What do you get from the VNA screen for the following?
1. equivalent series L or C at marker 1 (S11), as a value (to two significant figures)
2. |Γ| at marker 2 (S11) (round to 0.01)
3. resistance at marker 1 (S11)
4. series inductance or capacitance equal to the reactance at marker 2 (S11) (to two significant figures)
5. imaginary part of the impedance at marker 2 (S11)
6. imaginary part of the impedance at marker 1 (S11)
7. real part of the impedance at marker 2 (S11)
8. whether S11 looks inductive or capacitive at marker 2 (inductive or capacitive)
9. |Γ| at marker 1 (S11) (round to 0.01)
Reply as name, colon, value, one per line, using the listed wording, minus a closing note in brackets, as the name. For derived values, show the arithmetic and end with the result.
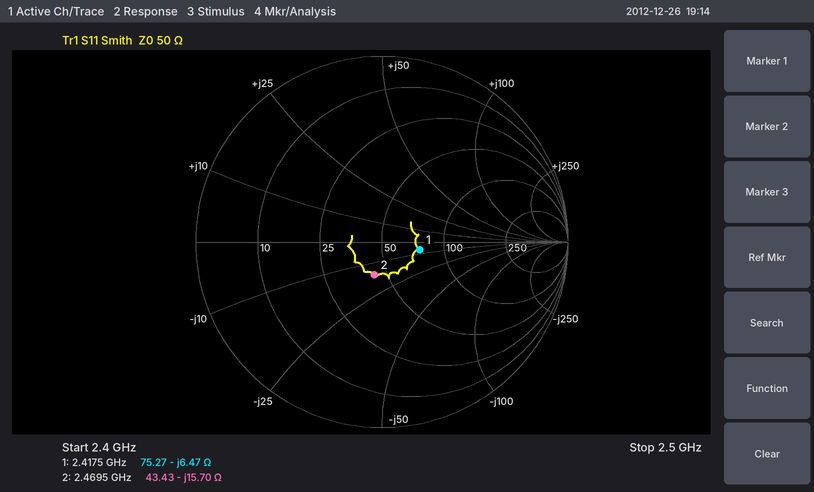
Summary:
equivalent series L or C at marker 1 (S11), as a value: C = 1/(2π × 2.4175 GHz × 6.47 Ω) ≈ 10 pF
|Γ| at marker 2 (S11): 0.18
resistance at marker 1: 75.27 Ω
series inductance or capacitance equal to the reactance at marker 2 (S11): C = 1/(2π × 2.4695 GHz × 15.7 Ω) ≈ 4.1 pF
imaginary part of the impedance at marker 2: -15.70 Ω
imaginary part of the impedance at marker 1: -6.47 Ω
real part of the impedance at marker 2: 43.43 Ω
whether S11 looks inductive or capacitive at marker 2: capacitive
|Γ| at marker 1 (S11): 0.21
